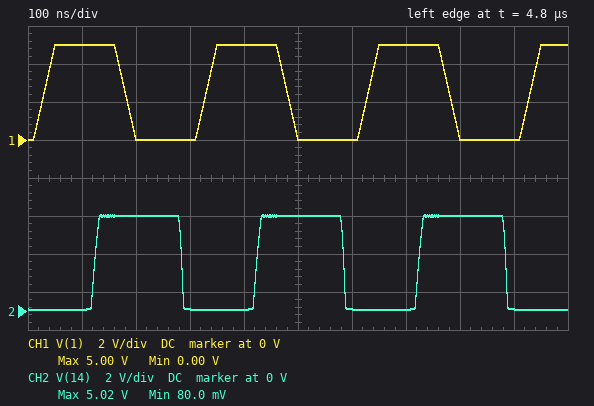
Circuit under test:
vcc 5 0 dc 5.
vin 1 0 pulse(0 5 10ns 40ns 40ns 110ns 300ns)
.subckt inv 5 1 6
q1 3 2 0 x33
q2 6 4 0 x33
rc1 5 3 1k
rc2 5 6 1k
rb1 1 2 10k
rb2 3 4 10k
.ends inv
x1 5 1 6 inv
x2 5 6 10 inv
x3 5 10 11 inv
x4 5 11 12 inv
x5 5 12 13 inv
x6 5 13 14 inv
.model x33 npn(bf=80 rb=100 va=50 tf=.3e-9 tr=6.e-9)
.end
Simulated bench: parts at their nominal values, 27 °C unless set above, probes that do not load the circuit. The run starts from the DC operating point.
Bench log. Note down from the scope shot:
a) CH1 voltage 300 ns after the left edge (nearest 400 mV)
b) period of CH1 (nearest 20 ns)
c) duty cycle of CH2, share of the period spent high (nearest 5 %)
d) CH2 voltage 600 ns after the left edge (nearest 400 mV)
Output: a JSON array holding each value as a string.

["0 V", "300 ns", "55 %", "0 V"]
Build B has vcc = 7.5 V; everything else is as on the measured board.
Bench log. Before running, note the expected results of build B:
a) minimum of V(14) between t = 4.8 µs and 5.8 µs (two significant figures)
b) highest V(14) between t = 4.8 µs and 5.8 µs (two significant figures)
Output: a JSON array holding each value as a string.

["74 mV", "7.5 V"]
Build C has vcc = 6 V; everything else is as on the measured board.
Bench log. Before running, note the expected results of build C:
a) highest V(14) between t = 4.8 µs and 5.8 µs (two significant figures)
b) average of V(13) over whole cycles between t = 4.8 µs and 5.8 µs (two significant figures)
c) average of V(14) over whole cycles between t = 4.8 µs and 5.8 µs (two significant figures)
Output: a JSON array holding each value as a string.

["6.0 V", "2.9 V", "3.2 V"]
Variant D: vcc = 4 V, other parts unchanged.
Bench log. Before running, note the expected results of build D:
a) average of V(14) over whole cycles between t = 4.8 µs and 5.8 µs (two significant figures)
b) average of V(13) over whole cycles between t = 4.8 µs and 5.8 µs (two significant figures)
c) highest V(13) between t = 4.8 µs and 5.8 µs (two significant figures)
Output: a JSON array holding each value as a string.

["2.2 V", "2.1 V", "3.7 V"]
